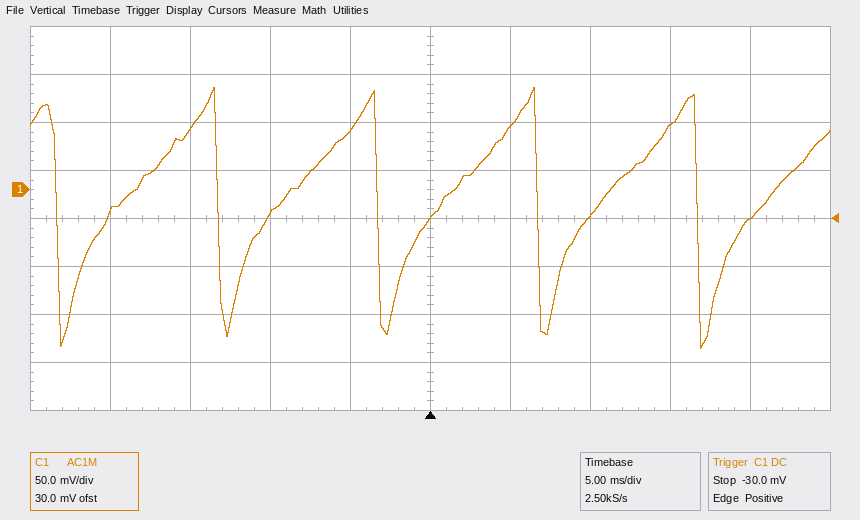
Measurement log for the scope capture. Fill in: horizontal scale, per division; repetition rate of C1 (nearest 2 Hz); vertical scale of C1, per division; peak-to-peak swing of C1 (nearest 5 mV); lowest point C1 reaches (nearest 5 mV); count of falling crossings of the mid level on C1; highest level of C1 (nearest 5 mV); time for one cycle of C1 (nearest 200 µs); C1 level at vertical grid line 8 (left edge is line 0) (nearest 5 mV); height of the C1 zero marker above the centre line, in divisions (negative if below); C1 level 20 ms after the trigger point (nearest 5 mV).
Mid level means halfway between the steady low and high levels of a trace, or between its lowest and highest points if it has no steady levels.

5 ms
100 Hz
50 mV
270 mV
-165 mV
5
105 mV
10.0 ms
65 mV
+0.6 div
-30 mV
